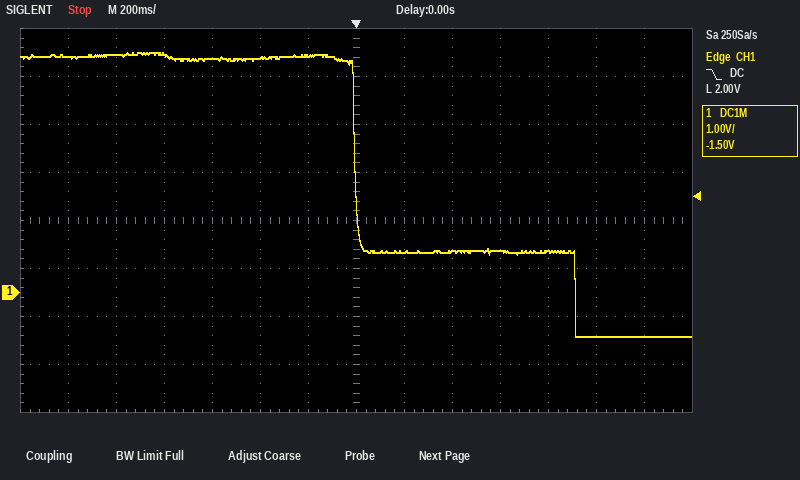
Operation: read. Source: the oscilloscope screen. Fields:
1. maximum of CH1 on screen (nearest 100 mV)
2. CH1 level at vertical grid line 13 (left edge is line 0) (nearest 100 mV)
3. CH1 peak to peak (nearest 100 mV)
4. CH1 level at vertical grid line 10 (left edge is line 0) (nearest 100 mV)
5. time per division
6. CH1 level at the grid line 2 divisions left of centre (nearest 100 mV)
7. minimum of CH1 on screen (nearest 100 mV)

5.0 V
-900 mV
5.9 V
900 mV
200 ms
4.9 V
-900 mV
